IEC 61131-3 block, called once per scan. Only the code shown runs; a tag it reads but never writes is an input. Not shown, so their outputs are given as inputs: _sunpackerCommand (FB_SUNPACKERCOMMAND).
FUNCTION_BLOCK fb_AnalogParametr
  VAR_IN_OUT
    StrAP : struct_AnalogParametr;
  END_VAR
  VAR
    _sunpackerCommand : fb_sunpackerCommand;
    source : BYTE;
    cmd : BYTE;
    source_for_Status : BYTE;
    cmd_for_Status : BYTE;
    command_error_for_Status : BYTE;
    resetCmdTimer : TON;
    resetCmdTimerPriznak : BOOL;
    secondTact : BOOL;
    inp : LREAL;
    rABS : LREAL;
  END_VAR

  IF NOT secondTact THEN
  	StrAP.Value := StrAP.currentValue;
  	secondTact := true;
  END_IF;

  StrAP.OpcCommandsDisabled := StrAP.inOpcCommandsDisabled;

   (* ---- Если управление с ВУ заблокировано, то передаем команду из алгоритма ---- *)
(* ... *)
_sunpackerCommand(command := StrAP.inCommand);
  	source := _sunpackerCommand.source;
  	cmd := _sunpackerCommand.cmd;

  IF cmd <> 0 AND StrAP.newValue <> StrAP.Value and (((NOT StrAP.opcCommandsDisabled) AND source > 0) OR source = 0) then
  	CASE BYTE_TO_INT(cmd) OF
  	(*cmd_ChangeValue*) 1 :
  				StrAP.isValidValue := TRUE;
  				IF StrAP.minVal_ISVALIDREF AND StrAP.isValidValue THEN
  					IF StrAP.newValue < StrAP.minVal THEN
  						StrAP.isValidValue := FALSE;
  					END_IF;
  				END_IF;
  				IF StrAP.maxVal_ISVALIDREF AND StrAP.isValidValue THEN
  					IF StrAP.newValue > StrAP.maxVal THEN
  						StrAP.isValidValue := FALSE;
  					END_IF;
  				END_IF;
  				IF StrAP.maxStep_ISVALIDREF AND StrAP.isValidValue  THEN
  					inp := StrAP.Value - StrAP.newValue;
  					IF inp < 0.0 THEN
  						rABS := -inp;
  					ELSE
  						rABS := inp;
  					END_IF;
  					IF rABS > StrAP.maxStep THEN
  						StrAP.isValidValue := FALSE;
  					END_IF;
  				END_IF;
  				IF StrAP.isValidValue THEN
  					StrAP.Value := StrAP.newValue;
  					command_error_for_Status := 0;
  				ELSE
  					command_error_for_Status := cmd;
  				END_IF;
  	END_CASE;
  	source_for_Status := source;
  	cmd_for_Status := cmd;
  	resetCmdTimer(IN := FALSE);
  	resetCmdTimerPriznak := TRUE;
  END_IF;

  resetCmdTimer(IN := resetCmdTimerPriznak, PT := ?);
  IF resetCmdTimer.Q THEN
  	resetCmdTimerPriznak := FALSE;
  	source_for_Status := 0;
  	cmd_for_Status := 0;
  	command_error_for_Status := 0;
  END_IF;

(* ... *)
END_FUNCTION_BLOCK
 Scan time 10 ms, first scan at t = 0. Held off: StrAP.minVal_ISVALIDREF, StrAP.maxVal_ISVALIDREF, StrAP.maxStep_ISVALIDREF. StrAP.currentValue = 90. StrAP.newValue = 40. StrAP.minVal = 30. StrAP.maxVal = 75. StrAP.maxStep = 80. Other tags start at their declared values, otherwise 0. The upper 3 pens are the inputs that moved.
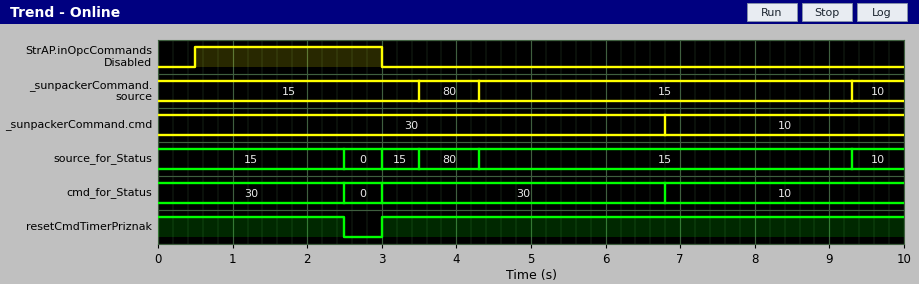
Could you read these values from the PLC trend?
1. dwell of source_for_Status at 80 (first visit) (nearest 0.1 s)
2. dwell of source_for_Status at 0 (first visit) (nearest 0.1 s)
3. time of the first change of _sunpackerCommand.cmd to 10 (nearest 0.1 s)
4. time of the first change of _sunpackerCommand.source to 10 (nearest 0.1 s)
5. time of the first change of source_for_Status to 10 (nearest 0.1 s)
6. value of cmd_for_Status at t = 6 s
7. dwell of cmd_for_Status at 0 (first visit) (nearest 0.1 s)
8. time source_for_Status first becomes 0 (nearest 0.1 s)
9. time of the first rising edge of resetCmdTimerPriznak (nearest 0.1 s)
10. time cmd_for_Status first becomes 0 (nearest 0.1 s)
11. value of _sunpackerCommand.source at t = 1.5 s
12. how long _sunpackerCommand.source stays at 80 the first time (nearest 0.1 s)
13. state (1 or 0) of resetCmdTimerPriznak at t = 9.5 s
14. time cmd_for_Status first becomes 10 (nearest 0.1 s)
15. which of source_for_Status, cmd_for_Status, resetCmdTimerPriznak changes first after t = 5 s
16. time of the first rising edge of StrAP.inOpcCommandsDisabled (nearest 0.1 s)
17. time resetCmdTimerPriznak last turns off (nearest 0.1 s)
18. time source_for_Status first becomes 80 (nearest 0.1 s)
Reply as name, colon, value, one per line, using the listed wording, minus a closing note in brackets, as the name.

dwell of source_for_Status at 80 (first visit): 0.8 s
dwell of source_for_Status at 0 (first visit): 0.5 s
time of the first change of _sunpackerCommand.cmd to 10: 6.8 s
time of the first change of _sunpackerCommand.source to 10: 9.3 s
time of the first change of source_for_Status to 10: 9.3 s
value of cmd_for_Status at t = 6 s: 30
dwell of cmd_for_Status at 0 (first visit): 0.5 s
time source_for_Status first becomes 0: 2.5 s
time of the first rising edge of resetCmdTimerPriznak: 3.0 s
time cmd_for_Status first becomes 0: 2.5 s
value of _sunpackerCommand.source at t = 1.5 s: 15
how long _sunpackerCommand.source stays at 80 the first time: 0.8 s
state (1 or 0) of resetCmdTimerPriznak at t = 9.5 s: 1
time cmd_for_Status first becomes 10: 6.8 s
which of source_for_Status, cmd_for_Status, resetCmdTimerPriznak changes first after t = 5 s: cmd_for_Status
time of the first rising edge of StrAP.inOpcCommandsDisabled: 0.5 s
time resetCmdTimerPriznak last turns off: 2.5 s
time source_for_Status first becomes 80: 3.5 s
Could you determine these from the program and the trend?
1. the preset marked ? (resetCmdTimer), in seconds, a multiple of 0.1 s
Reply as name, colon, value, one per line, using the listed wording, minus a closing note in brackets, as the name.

the preset marked ? (resetCmdTimer), in seconds, a multiple of 0.1 s: 2.0 s
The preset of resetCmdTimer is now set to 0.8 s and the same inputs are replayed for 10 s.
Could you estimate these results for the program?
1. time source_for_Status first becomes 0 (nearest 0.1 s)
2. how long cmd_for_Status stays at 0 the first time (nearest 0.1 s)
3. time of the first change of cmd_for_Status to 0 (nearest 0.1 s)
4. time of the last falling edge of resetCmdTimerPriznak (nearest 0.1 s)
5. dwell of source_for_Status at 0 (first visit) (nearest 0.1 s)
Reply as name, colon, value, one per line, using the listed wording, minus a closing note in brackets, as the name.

time source_for_Status first becomes 0: 1.3 s
how long cmd_for_Status stays at 0 the first time: 1.7 s
time of the first change of cmd_for_Status to 0: 1.3 s
time of the last falling edge of resetCmdTimerPriznak: 1.3 s
dwell of source_for_Status at 0 (first visit): 1.7 s
